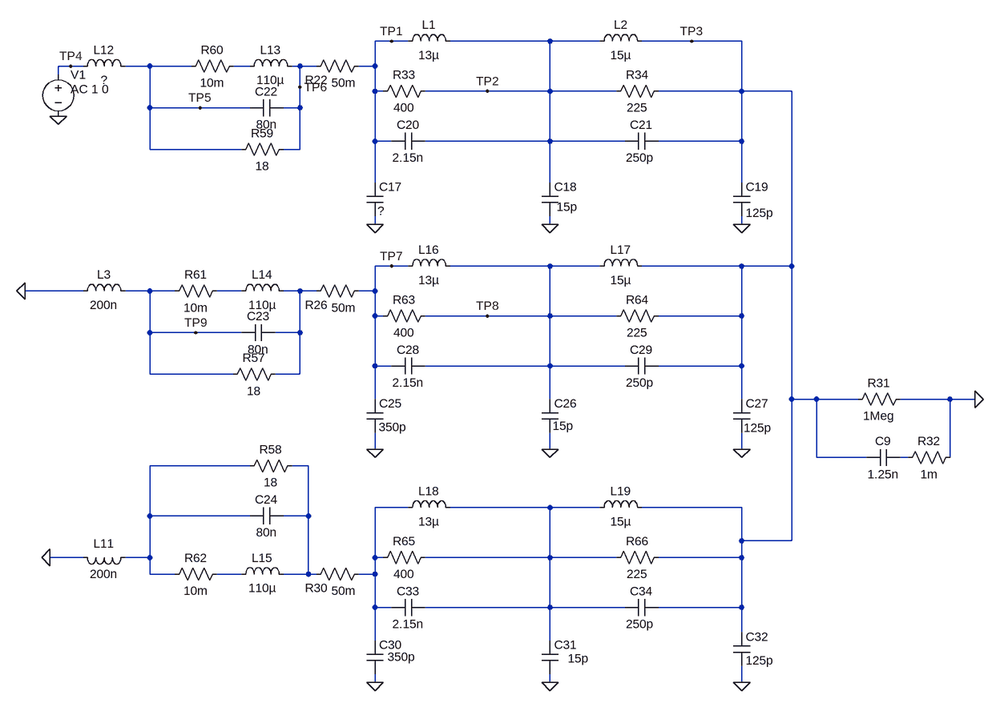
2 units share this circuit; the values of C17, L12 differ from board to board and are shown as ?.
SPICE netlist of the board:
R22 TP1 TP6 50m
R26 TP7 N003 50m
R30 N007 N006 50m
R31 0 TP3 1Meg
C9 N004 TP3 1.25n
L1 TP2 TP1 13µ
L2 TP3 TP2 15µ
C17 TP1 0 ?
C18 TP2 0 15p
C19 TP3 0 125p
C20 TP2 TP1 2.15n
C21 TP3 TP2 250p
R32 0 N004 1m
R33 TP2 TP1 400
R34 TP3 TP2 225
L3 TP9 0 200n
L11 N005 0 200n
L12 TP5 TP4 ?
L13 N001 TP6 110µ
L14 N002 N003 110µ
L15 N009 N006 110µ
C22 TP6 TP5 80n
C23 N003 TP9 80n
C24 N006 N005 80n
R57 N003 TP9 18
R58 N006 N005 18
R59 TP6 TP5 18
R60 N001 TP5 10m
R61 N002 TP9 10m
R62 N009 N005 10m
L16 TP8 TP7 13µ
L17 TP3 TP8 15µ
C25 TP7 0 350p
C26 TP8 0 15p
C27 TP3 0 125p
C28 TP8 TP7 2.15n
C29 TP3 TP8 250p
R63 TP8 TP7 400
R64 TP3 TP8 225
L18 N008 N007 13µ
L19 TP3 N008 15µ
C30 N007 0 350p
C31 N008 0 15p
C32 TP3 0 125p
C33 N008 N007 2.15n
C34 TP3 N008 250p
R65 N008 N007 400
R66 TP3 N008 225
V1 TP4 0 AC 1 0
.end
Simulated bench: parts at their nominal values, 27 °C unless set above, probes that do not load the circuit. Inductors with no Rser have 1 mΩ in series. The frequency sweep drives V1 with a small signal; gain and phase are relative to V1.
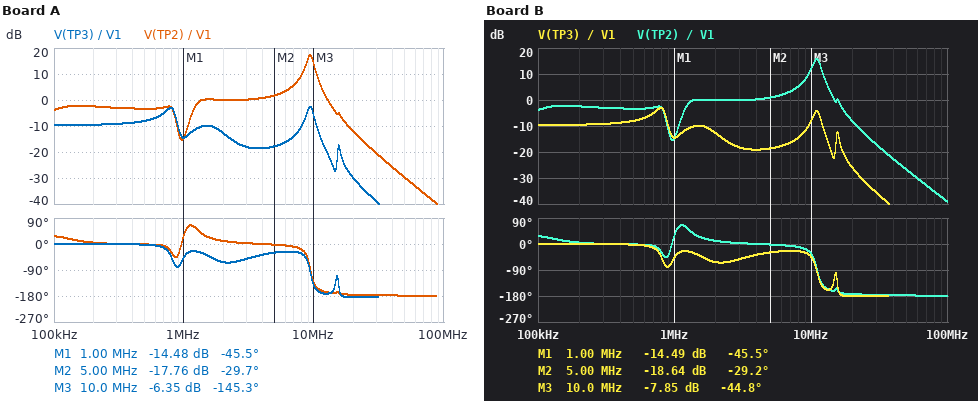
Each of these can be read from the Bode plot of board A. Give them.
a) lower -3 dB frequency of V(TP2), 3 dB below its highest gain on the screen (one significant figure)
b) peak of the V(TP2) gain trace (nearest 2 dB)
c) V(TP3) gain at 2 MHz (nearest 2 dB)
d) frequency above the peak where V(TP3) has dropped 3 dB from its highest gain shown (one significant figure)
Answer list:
9 MHz
18 dB
-12 dB
10 MHz
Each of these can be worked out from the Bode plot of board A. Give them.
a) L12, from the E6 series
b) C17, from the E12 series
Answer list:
680 nH
220 pF
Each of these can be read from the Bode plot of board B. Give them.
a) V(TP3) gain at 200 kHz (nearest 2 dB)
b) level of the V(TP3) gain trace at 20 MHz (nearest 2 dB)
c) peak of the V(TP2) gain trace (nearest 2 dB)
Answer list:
-10 dB
-26 dB
16 dB
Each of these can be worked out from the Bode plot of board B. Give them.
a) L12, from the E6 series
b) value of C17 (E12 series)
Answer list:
680 nH
100 pF
